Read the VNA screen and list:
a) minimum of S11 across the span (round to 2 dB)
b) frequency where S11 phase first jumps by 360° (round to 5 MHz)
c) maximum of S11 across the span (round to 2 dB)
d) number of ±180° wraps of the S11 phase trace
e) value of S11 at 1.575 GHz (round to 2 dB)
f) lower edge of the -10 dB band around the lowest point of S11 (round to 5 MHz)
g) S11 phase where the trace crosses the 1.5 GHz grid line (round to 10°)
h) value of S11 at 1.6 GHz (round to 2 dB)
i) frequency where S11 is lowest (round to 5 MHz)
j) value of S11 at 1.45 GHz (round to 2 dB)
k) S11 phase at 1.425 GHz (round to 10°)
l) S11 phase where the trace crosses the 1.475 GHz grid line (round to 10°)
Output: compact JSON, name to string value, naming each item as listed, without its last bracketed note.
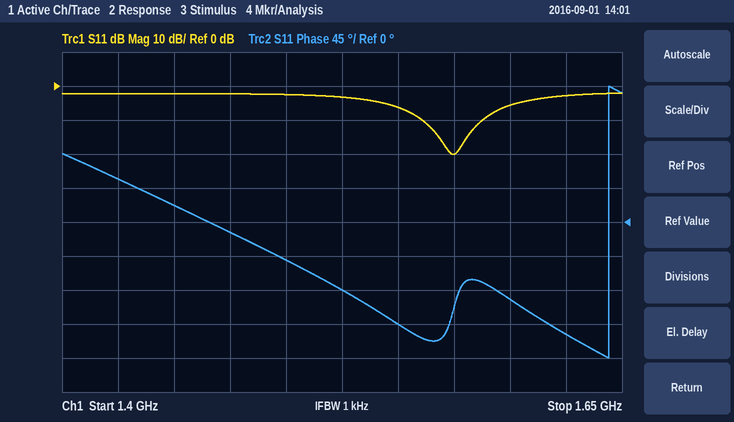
{"minimum of S11 across the span": "-20 dB", "frequency where S11 phase first jumps by 360°": "1.645 GHz", "maximum of S11 across the span": "-2 dB", "number of ±180° wraps of the S11 phase trace": "1", "value of S11 at 1.575 GHz": "-20 dB", "lower edge of the -10 dB band around the lowest point of S11": "1.560 GHz", "S11 phase where the trace crosses the 1.5 GHz grid line": "-50°", "value of S11 at 1.6 GHz": "-6 dB", "frequency where S11 is lowest": "1.575 GHz", "value of S11 at 1.45 GHz": "-2 dB", "S11 phase at 1.425 GHz": "60°", "S11 phase where the trace crosses the 1.475 GHz grid line": "-10°"}
